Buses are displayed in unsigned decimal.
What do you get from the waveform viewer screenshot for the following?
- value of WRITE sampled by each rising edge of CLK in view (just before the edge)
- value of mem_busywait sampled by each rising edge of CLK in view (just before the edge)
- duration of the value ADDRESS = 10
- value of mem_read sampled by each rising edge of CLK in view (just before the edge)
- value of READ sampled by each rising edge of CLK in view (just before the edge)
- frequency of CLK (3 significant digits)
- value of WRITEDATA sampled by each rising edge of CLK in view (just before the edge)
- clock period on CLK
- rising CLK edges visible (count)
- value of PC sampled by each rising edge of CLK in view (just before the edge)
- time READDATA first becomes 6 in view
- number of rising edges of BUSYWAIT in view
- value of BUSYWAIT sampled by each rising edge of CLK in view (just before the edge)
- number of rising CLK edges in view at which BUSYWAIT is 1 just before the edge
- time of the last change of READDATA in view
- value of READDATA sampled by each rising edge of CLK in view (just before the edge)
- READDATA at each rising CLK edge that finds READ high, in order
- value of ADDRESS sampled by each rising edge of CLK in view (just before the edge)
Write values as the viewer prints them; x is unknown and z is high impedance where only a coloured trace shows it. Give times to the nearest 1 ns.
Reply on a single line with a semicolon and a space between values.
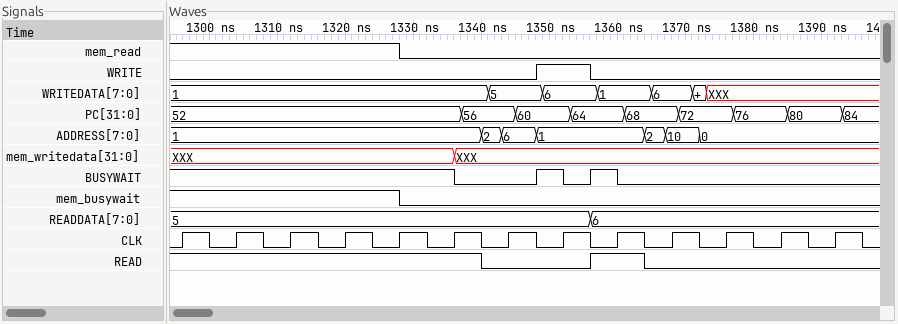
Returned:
0 0 0 0 0 0 0 1 0 0 0 0 0; 1 1 1 1 1 0 0 0 0 0 0 0 0; 5 ns; 1 1 1 1 1 0 0 0 0 0 0 0 0; 1 1 1 1 1 1 0 0 1 0 0 0 0; 125 MHz; 1, 1, 1, 1, 1, 1, 5, 6, 1, 6, XXX, XXX, XXX; 8 ns; 13; 52, 52, 52, 52, 52, 52, 56, 60, 64, 68, 72, 76, 80; 1356 ns; 2; 1 1 1 1 1 1 0 1 1 0 0 0 0; 8; 1356 ns; 5, 5, 5, 5, 5, 5, 5, 5, 6, 6, 6, 6, 6; 5, 5, 5, 5, 5, 5, 6; 1, 1, 1, 1, 1, 1, 6, 1, 1, 10, 0, 0, 0
